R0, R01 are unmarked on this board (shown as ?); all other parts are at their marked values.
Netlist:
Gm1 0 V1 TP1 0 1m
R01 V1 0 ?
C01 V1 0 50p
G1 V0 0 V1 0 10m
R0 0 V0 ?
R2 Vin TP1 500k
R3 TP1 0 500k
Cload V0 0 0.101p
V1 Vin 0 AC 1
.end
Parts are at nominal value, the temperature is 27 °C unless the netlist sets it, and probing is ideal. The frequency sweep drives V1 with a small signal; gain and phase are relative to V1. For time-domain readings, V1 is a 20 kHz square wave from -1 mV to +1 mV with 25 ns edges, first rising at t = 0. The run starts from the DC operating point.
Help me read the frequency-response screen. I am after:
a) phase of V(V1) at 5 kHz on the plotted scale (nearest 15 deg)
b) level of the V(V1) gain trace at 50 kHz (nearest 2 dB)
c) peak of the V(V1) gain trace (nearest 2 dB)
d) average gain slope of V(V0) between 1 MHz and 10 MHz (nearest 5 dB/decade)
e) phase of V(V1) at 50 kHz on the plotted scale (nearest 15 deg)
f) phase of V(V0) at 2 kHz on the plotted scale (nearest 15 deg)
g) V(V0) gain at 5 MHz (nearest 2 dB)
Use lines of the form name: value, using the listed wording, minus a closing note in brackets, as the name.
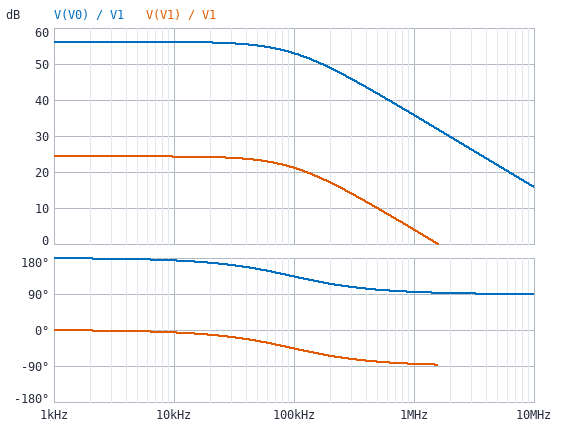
phase of V(V1) at 5 kHz on the plotted scale: 0 deg
level of the V(V1) gain trace at 50 kHz: 24 dB
peak of the V(V1) gain trace: 24 dB
average gain slope of V(V0) between 1 MHz and 10 MHz: -20 dB/decade
phase of V(V1) at 50 kHz on the plotted scale: -30 deg
phase of V(V0) at 2 kHz on the plotted scale: 180 deg
V(V0) gain at 5 MHz: 22 dB
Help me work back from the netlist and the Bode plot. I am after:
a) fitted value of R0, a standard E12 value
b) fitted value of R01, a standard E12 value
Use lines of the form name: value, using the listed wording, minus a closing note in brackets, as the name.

fitted value of R0, a standard E12 value: 3.9 kΩ
fitted value of R01, a standard E12 value: 33 kΩ
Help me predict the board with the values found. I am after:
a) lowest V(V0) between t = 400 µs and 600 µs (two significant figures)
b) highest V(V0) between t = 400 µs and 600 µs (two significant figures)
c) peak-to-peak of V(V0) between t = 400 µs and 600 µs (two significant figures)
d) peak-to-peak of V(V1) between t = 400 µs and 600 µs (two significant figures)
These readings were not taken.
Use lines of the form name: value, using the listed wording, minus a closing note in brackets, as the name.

lowest V(V0) between t = 400 µs and 600 µs: -640 mV
highest V(V0) between t = 400 µs and 600 µs: 640 mV
peak-to-peak of V(V0) between t = 400 µs and 600 µs: 1.3 V
peak-to-peak of V(V1) between t = 400 µs and 600 µs: 33 mV
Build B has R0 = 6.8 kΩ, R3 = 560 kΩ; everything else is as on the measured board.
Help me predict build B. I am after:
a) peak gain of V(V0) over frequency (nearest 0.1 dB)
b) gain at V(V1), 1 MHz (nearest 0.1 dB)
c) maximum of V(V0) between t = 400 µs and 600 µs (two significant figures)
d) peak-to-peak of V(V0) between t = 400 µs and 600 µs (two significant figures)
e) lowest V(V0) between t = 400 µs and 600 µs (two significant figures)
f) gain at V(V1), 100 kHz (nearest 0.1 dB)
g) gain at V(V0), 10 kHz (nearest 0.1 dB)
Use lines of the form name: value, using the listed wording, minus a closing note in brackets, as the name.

peak gain of V(V0) over frequency: 61.5 dB
gain at V(V1), 1 MHz: 4.5 dB
maximum of V(V0) between t = 400 µs and 600 µs: 1.2 V
peak-to-peak of V(V0) between t = 400 µs and 600 µs: 2.4 V
lowest V(V0) between t = 400 µs and 600 µs: -1.2 V
gain at V(V1), 100 kHz: 21.7 dB
gain at V(V0), 10 kHz: 61.4 dB
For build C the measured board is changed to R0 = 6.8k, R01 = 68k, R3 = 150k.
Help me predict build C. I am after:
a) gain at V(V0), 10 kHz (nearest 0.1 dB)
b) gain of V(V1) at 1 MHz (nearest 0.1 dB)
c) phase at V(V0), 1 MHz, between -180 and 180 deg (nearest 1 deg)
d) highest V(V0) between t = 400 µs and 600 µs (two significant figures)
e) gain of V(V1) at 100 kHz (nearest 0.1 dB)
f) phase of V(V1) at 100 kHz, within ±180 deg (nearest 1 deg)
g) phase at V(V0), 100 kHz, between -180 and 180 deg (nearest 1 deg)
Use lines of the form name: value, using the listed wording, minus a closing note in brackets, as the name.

gain at V(V0), 10 kHz: 60.4 dB
gain of V(V1) at 1 MHz: -2.7 dB
phase at V(V0), 1 MHz, between -180 and 180 deg: 92 deg
highest V(V0) between t = 400 µs and 600 µs: 1.1 V
gain of V(V1) at 100 kHz: 16.5 dB
phase of V(V1) at 100 kHz, within ±180 deg: -65 deg
phase at V(V0), 100 kHz, between -180 and 180 deg: 115 deg
